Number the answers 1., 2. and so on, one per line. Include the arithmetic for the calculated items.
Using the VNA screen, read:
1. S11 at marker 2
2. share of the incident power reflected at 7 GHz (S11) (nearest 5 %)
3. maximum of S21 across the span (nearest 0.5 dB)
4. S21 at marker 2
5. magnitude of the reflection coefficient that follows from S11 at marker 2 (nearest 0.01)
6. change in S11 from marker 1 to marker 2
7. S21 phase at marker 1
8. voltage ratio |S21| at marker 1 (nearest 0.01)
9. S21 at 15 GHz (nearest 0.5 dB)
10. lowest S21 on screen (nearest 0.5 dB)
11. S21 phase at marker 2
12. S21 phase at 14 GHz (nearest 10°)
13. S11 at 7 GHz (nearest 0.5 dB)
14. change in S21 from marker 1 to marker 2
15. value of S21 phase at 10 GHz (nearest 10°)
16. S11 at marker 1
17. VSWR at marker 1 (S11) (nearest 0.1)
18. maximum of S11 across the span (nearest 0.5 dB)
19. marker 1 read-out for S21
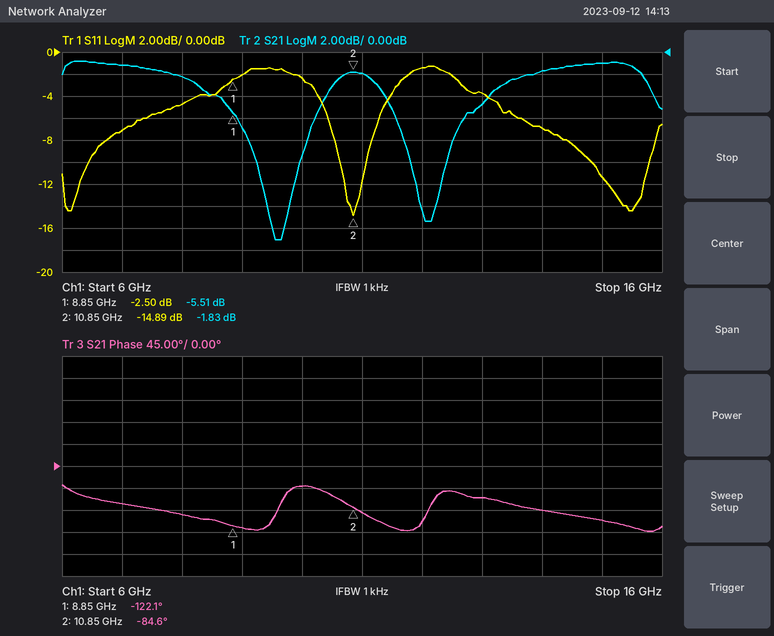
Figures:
1. -14.89 dB
2. 10^(-7/10) ≈ 20 %
3. -1.0 dB
4. -1.83 dB
5. 10^(-14.89/20) ≈ 0.18
6. -14.89 − (-2.5) = -12.39 dB
7. -122.1°
8. 10^(-5.51/20) ≈ 0.53
9. -1.0 dB
10. -17.0 dB
11. -84.6°
12. -90°
13. -7.0 dB
14. -1.83 − (-5.51) = 3.68 dB
15. -40°
16. -2.50 dB
17. (1 + 0.7499)/(1 − 0.7499) ≈ 7.0
18. -1.5 dB
19. -5.51 dB
